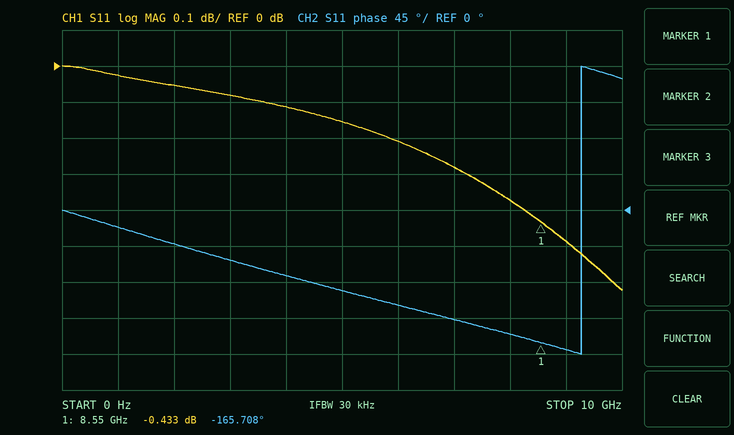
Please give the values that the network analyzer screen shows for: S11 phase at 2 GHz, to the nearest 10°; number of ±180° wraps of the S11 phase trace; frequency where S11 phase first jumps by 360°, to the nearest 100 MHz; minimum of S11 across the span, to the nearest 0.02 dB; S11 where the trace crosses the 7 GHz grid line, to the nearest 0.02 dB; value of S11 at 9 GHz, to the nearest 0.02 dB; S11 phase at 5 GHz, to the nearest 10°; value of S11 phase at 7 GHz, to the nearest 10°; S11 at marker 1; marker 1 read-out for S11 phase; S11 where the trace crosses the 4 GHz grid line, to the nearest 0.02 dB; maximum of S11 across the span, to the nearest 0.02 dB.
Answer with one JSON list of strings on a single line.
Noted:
["-40°", "1", "9.3 GHz", "-0.62 dB", "-0.28 dB", "-0.48 dB", "-100°", "-140°", "-0.433 dB", "-165.708°", "-0.12 dB", "0.00 dB"]
